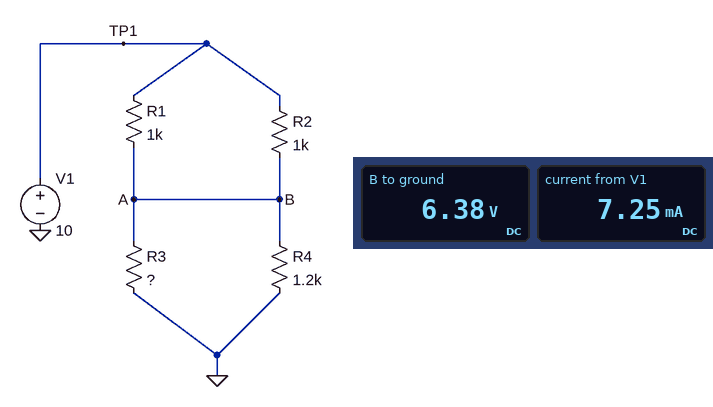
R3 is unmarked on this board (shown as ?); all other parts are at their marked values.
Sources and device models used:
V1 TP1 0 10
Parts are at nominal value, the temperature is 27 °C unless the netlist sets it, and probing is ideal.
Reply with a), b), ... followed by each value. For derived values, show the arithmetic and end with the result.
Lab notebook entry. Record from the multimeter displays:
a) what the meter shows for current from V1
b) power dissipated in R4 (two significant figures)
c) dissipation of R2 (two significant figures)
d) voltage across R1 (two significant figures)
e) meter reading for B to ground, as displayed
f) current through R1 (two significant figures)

a) 7.25 mA
b) (6.38 V)^2 / 1.2 kΩ = 34 mW
c) (10 V - 6.38 V)^2 / 1 kΩ = 13 mW
d) 10 V - 6.38 V = 3.6 V
e) 6.38 V
f) (10 V - 6.38 V) / 1 kΩ = 3.6 mA
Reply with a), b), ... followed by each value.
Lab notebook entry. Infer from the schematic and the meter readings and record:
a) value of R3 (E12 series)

a) 3.3 kΩ
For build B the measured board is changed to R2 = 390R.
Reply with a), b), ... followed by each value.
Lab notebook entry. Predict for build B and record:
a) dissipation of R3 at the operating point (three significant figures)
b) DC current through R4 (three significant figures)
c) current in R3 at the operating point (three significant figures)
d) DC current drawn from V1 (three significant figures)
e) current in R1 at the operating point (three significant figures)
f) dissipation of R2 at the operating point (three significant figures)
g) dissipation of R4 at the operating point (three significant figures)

a) 17.4 mW
b) 6.32 mA
c) 2.30 mA
d) 8.62 mA
e) 2.42 mA
f) 15.0 mW
g) 47.9 mW
